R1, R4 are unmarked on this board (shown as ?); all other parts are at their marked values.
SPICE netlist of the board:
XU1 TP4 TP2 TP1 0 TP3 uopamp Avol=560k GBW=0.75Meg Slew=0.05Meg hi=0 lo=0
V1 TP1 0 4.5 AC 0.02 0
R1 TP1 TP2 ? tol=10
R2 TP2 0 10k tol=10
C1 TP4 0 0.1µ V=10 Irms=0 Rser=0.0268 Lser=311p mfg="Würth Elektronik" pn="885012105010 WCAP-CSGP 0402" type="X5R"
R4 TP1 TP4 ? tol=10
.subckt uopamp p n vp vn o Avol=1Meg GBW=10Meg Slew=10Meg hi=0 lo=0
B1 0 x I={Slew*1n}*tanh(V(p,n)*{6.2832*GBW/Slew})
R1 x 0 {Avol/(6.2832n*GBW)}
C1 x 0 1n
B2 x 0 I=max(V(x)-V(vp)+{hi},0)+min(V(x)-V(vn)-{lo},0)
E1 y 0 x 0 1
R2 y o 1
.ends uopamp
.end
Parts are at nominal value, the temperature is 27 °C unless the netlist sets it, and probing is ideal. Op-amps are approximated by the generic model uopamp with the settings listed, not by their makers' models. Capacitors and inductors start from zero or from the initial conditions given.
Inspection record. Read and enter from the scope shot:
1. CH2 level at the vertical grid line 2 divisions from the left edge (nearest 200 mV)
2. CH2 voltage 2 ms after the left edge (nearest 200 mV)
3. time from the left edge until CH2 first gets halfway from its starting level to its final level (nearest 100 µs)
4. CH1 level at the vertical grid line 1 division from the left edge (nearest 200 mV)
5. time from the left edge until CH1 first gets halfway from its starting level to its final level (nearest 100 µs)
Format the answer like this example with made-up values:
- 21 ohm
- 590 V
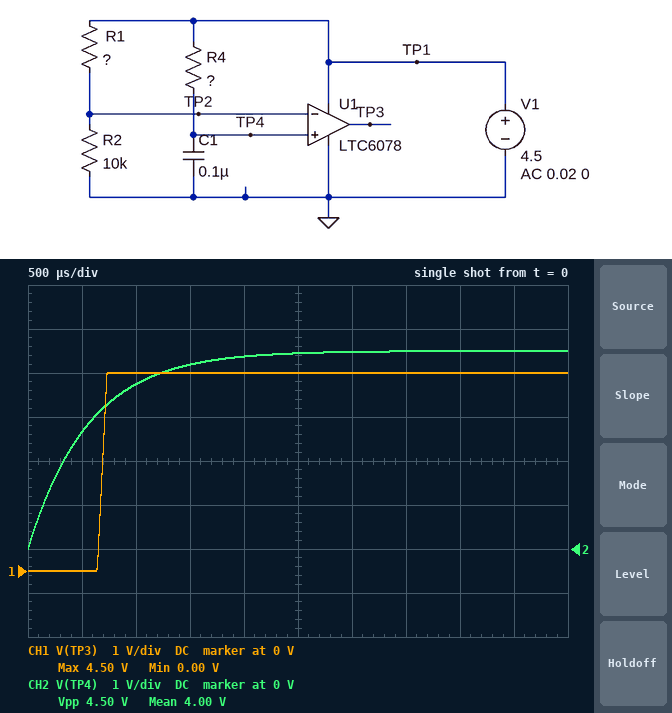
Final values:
- 3.8 V
- 4.4 V
- 400 µs
- 0 V
- 700 µs
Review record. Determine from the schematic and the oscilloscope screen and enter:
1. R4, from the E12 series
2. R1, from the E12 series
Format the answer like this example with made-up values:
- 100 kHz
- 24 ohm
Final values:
- 5.6 kΩ
- 4.7 kΩ
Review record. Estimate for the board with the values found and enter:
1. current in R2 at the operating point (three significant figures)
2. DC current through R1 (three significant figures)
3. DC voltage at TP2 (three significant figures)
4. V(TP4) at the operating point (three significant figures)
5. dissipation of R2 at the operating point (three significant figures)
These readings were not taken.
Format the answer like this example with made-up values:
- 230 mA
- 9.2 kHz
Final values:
- 306 µA
- 306 µA
- 3.06 V
- 4.50 V
- 937 µW
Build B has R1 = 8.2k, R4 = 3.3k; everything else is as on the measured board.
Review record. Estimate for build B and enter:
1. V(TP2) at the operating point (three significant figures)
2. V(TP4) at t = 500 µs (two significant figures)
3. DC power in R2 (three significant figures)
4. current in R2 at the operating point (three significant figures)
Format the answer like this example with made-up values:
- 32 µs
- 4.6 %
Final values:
- 2.47 V
- 3.5 V
- 611 µW
- 247 µA
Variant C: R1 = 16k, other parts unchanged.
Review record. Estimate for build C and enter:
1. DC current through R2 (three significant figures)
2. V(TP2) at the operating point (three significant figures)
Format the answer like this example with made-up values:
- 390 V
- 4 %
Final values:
- 173 µA
- 1.73 V
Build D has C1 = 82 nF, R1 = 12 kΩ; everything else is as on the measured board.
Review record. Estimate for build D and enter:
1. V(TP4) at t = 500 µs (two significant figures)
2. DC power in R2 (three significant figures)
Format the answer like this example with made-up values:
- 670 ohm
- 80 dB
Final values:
- 3.0 V
- 418 µW
